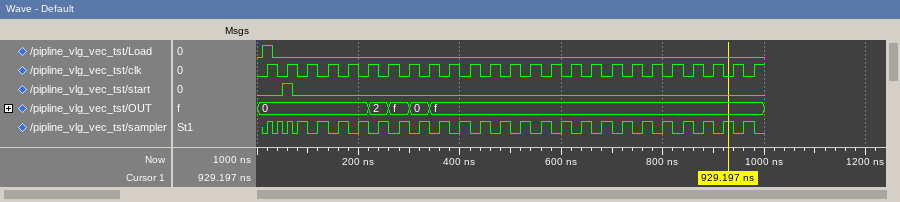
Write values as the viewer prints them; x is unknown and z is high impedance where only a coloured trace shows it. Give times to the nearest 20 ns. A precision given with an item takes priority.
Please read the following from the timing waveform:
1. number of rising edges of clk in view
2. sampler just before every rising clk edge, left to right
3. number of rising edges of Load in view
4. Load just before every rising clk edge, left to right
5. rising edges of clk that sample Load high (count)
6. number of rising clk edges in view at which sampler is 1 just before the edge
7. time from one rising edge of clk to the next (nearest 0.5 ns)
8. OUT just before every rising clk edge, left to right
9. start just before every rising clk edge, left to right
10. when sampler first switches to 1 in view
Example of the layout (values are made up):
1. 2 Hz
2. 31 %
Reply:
1. 25
2. 0 0 1 1 1 1 1 1 1 1 1 1 1 1 1 1 1 1 1 1 1 1 1 1 1
3. 1
4. 1 0 0 0 0 0 0 0 0 0 0 0 0 0 0 0 0 0 0 0 0 0 0 0 0
5. 1
6. 23
7. 40 ns
8. 0, 0, 0, 0, 0, 0, 2, f, 0, f, f, f, f, f, f, f, f, f, f, f, f, f, f, f, f
9. 0 1 0 0 0 0 0 0 0 0 0 0 0 0 0 0 0 0 0 0 0 0 0 0 0
10. 20 ns
